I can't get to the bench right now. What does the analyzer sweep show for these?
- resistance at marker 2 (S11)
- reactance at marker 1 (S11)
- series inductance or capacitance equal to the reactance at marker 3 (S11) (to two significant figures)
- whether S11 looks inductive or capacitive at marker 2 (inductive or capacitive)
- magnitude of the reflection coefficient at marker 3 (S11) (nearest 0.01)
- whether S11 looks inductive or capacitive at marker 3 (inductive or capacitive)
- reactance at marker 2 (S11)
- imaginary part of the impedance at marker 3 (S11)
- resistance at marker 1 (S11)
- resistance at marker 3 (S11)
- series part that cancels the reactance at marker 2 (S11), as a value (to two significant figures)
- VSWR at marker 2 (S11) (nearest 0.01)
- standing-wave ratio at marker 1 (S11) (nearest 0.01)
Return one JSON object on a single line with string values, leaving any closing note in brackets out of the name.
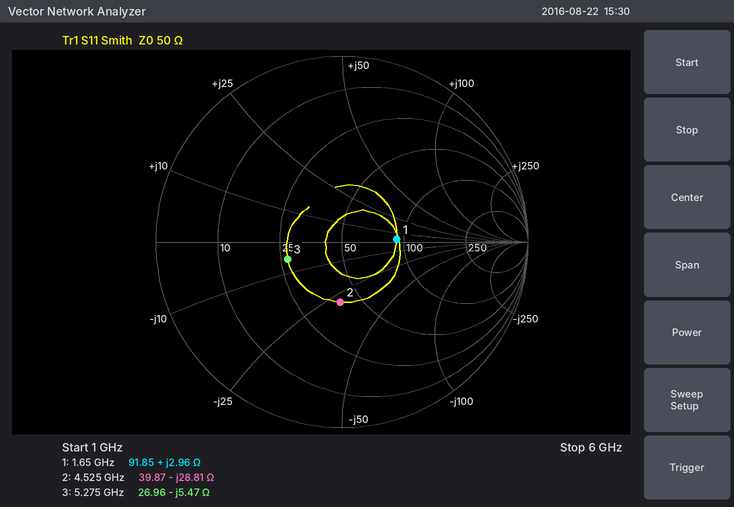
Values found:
{"resistance at marker 2": "39.87 Ω", "reactance at marker 1": "+2.96 Ω", "series inductance or capacitance equal to the reactance at marker 3 (S11)": "5.5 pF", "whether S11 looks inductive or capacitive at marker 2": "capacitive", "magnitude of the reflection coefficient at marker 3 (S11)": "0.31", "whether S11 looks inductive or capacitive at marker 3": "capacitive", "reactance at marker 2": "-28.81 Ω", "imaginary part of the impedance at marker 3": "-5.47 Ω", "resistance at marker 1": "91.85 Ω", "resistance at marker 3": "26.96 Ω", "series part that cancels the reactance at marker 2 (S11), as a value": "1.0 nH", "VSWR at marker 2 (S11)": "1.96", "standing-wave ratio at marker 1 (S11)": "1.84"}
